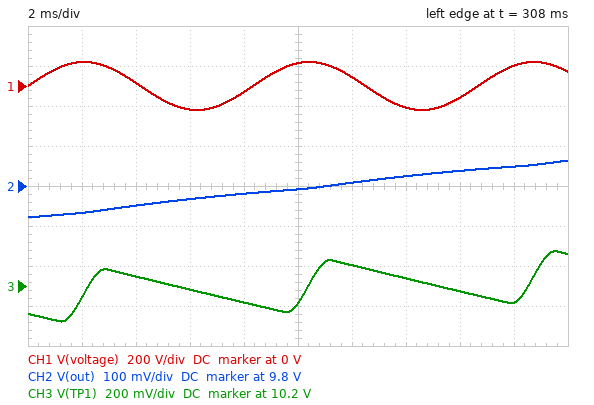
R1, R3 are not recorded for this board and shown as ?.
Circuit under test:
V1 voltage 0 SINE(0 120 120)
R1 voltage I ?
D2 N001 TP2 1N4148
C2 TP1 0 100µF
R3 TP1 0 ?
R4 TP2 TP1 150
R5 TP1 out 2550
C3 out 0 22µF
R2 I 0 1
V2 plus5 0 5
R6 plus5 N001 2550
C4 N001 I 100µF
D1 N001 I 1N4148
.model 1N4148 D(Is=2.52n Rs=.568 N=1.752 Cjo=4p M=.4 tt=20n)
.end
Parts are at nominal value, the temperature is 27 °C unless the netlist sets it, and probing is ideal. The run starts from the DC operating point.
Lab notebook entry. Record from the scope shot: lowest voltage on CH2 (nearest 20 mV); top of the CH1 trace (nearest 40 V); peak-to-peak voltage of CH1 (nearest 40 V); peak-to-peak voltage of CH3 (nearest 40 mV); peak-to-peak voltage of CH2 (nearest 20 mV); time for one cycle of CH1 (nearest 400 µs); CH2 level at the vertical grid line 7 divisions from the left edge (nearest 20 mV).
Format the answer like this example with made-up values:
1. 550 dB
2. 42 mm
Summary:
1. 9.72 V
2. 120 V
3. 240 V
4. 360 mV
5. 140 mV
6. 8.4 ms
7. 9.82 V
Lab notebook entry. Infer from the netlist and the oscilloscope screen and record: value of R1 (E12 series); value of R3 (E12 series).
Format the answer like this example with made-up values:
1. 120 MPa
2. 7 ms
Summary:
1. 4.7 Ω
2. 3.3 kΩ
